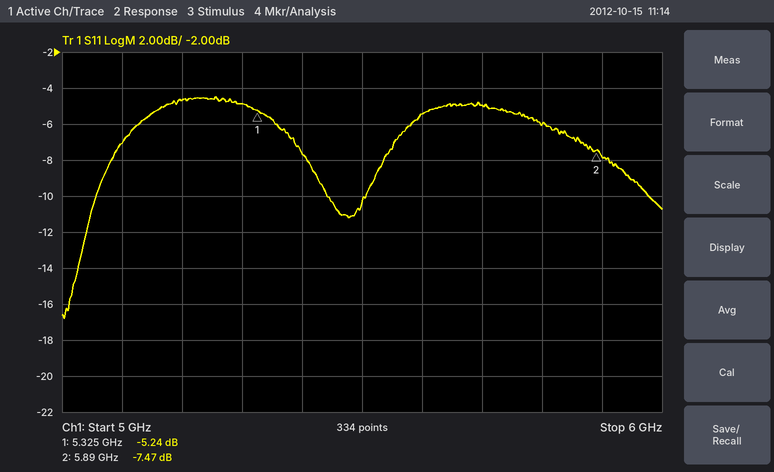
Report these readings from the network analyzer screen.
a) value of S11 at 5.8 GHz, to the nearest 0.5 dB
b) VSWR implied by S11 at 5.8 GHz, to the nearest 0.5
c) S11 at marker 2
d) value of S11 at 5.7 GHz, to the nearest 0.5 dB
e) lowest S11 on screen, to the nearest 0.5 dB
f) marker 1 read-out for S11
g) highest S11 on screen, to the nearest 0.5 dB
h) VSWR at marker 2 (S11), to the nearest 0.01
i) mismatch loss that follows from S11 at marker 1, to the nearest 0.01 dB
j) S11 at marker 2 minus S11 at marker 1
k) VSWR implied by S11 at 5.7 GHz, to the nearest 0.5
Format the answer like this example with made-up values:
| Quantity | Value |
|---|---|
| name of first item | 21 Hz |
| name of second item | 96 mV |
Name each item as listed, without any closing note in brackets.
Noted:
| Quantity | Value |
|---|---|
| value of S11 at 5.8 GHz, to the nearest 0.5 dB | -6.0 dB |
| VSWR implied by S11 at 5.8 GHz, to the nearest 0.5 | 3.0 |
| S11 at marker 2 | -7.47 dB |
| value of S11 at 5.7 GHz, to the nearest 0.5 dB | -5.0 dB |
| lowest S11 on screen, to the nearest 0.5 dB | -17.0 dB |
| marker 1 read-out for S11 | -5.24 dB |
| highest S11 on screen, to the nearest 0.5 dB | -4.5 dB |
| VSWR at marker 2 (S11), to the nearest 0.01 | 2.47 |
| mismatch loss that follows from S11 at marker 1, to the nearest 0.01 dB | 1.54 dB |
| S11 at marker 2 minus S11 at marker 1 | -2.23 dB |
| VSWR implied by S11 at 5.7 GHz, to the nearest 0.5 | 3.5 |
